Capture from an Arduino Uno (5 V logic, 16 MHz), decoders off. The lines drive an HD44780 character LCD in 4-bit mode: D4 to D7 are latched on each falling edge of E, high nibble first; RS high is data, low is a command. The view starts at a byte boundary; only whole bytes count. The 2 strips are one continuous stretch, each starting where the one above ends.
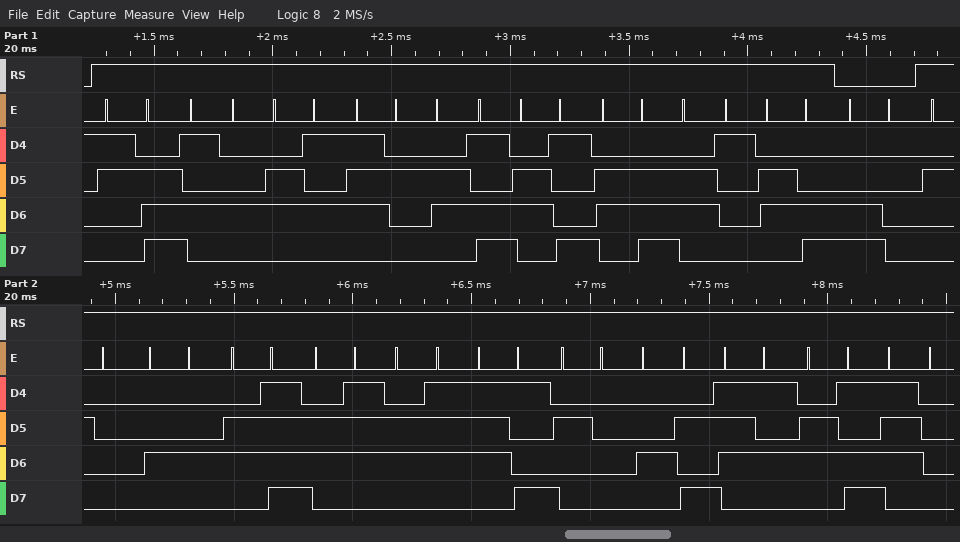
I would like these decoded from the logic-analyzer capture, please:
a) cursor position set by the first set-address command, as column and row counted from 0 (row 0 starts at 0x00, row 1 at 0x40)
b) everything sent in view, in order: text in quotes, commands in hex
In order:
column 0, row 1
">Terminal" 0xC0 " Doggy Jump"
